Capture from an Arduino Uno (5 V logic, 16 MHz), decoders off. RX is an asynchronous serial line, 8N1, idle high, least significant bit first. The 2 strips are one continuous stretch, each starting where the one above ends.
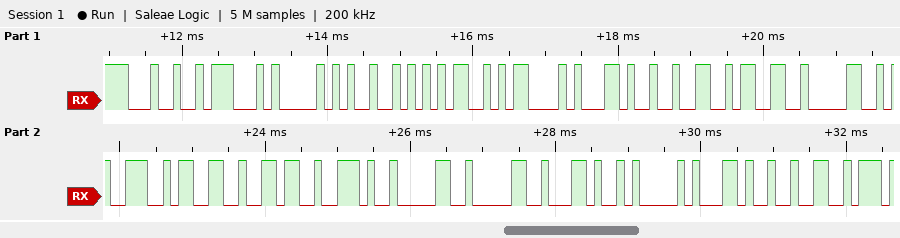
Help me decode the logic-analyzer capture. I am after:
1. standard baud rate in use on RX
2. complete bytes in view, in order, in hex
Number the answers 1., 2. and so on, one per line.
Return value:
1. 9600 baud
2. 0x24 0x47 0x50 0x52 0x4D 0x43 0x2C 0x32 0x33 0x30 0x39 0x33 0x36 0x2E 0x30 0x30 0x2C 0x41 0x2C 0x32
